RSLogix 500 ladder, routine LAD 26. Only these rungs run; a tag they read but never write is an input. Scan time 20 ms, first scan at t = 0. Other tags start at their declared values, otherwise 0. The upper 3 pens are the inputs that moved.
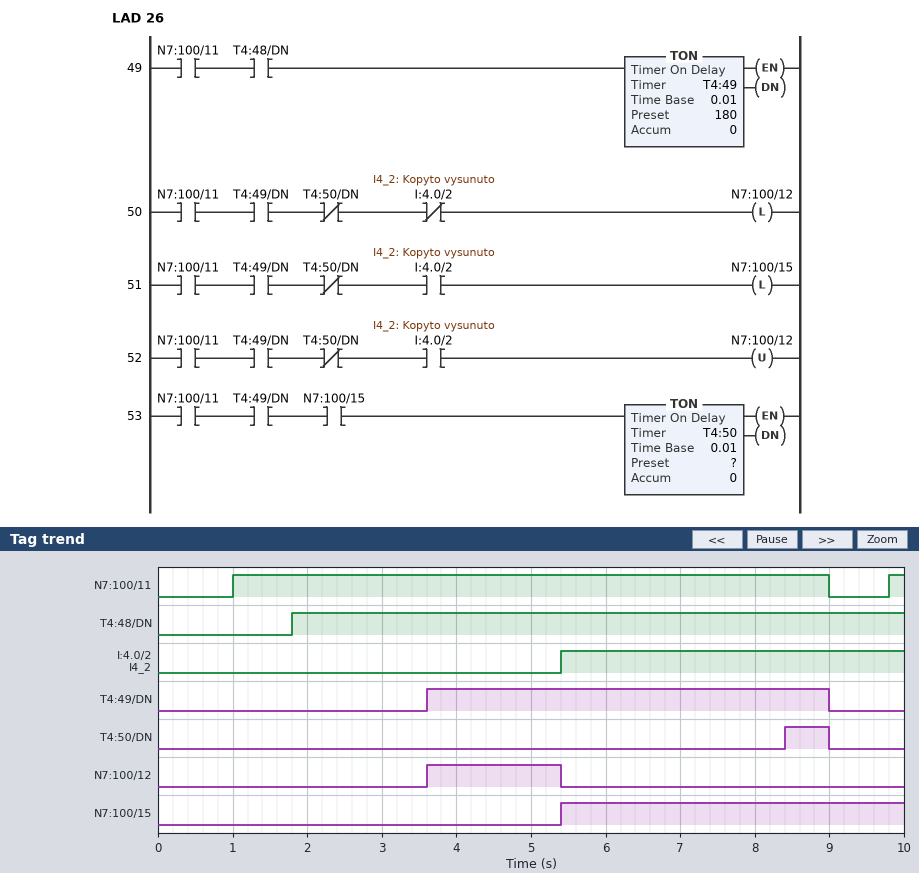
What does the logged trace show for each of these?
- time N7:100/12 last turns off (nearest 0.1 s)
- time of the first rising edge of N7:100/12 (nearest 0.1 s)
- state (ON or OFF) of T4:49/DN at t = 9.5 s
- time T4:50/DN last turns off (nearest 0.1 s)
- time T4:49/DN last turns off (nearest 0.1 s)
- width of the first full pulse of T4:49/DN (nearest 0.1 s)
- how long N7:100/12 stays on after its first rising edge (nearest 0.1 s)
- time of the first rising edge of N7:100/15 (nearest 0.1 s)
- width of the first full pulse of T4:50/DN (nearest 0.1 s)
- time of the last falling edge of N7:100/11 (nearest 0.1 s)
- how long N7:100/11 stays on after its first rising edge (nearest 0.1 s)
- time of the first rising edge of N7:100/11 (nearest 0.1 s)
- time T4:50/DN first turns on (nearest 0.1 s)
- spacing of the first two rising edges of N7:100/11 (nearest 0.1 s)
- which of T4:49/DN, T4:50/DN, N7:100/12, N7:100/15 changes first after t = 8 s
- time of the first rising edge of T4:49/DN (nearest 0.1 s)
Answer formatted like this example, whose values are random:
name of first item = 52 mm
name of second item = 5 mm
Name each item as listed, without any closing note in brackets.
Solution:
time N7:100/12 last turns off = 5.4 s
time of the first rising edge of N7:100/12 = 3.6 s
state (ON or OFF) of T4:49/DN at t = 9.5 s = OFF
time T4:50/DN last turns off = 9.0 s
time T4:49/DN last turns off = 9.0 s
width of the first full pulse of T4:49/DN = 5.4 s
how long N7:100/12 stays on after its first rising edge = 1.8 s
time of the first rising edge of N7:100/15 = 5.4 s
width of the first full pulse of T4:50/DN = 0.6 s
time of the last falling edge of N7:100/11 = 9.0 s
how long N7:100/11 stays on after its first rising edge = 8.0 s
time of the first rising edge of N7:100/11 = 1.0 s
time T4:50/DN first turns on = 8.4 s
spacing of the first two rising edges of N7:100/11 = 8.8 s
which of T4:49/DN, T4:50/DN, N7:100/12, N7:100/15 changes first after t = 8 s = T4:50/DN
time of the first rising edge of T4:49/DN = 3.6 s
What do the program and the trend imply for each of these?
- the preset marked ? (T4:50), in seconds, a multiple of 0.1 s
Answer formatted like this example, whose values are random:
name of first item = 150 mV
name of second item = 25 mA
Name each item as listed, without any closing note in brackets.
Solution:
the preset marked ? (T4:50), in seconds, a multiple of 0.1 s = 3.0 s
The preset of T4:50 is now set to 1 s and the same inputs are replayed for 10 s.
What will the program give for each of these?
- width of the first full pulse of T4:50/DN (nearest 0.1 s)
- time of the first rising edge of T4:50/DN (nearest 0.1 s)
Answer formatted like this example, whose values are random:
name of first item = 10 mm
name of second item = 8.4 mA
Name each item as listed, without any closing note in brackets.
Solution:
width of the first full pulse of T4:50/DN = 2.6 s
time of the first rising edge of T4:50/DN = 6.4 s
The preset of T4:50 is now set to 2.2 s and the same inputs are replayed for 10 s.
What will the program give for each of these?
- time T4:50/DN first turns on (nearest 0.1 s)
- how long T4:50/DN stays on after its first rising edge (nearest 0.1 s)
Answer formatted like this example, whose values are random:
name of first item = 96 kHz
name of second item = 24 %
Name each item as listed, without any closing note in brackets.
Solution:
time T4:50/DN first turns on = 7.6 s
how long T4:50/DN stays on after its first rising edge = 1.4 s
